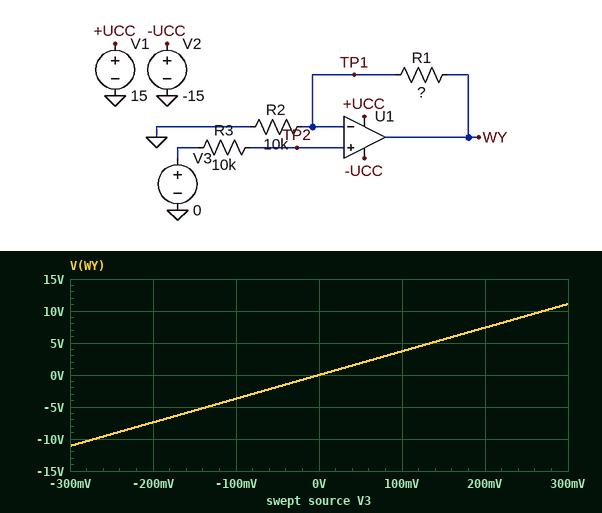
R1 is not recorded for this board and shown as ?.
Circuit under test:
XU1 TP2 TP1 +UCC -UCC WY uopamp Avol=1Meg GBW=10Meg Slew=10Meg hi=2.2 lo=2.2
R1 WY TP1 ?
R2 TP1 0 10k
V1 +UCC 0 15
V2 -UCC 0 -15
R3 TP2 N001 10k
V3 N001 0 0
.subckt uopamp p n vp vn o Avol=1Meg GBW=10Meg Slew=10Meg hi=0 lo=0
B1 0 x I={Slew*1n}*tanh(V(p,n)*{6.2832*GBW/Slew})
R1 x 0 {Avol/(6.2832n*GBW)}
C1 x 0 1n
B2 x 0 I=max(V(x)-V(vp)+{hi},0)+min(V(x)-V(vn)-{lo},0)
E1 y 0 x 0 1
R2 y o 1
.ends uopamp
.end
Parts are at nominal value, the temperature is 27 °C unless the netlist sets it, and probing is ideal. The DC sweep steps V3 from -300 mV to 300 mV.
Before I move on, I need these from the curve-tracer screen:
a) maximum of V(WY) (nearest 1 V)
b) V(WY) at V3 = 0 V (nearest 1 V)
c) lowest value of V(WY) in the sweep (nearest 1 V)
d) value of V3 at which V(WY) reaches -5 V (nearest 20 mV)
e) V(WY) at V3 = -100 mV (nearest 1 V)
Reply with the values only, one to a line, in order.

11 V
0 V
-11 V
-140 mV
-4 V
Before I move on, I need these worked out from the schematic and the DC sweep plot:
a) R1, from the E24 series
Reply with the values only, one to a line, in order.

360 kΩ
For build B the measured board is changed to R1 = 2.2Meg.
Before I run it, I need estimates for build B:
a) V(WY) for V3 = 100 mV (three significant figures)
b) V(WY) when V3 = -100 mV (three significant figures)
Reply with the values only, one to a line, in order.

12.8 V
-12.8 V
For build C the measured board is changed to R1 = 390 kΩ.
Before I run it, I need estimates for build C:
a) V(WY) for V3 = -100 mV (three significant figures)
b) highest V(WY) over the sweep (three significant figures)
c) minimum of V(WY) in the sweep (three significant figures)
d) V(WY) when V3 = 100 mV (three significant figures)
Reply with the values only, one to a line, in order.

-4.00 V
12.0 V
-12.0 V
4.00 V
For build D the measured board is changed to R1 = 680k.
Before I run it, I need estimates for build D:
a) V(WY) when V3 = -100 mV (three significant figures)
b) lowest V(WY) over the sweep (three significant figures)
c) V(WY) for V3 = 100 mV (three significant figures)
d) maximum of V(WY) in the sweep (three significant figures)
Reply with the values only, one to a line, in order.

-6.90 V
-12.8 V
6.90 V
12.8 V
